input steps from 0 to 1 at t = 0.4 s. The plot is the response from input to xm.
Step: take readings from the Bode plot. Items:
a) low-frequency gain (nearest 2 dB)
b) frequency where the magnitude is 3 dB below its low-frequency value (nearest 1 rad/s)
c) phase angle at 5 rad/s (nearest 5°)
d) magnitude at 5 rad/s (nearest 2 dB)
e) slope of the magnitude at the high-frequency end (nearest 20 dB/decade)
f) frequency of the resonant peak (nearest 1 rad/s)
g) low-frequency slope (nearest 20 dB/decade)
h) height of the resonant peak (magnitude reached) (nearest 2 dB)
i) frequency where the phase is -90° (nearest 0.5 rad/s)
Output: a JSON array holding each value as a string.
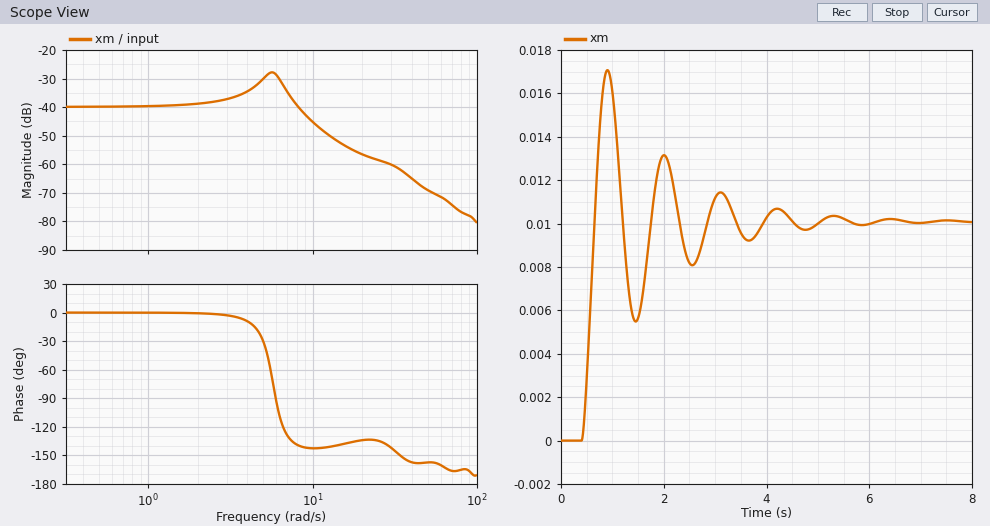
["-40 dB", "9 rad/s", "-30°", "-30 dB", "-40 dB/decade", "6 rad/s", "0 dB/decade", "-28 dB", "6.0 rad/s"]
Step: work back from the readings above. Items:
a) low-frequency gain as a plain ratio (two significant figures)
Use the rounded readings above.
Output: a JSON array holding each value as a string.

["0.010"]
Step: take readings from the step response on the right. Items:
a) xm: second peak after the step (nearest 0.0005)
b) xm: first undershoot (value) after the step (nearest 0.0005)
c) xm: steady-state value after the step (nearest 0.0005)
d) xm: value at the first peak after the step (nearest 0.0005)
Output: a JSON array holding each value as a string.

["0.0130", "0.0055", "0.0100", "0.0170"]
